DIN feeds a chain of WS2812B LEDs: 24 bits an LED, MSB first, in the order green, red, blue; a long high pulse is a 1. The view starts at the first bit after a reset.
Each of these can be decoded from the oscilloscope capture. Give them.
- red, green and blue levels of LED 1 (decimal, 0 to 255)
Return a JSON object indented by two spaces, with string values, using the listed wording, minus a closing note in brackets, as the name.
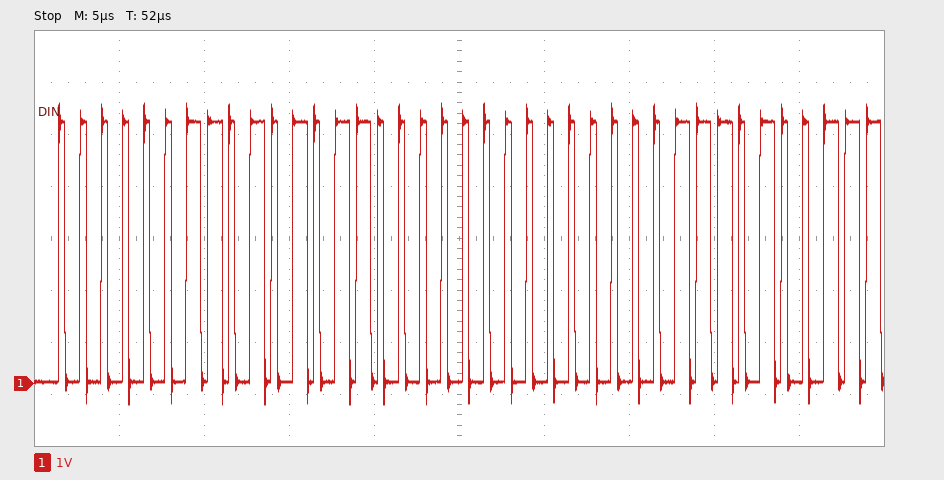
{
  "red, green and blue levels of LED 1": "86, 3, 0"
}
